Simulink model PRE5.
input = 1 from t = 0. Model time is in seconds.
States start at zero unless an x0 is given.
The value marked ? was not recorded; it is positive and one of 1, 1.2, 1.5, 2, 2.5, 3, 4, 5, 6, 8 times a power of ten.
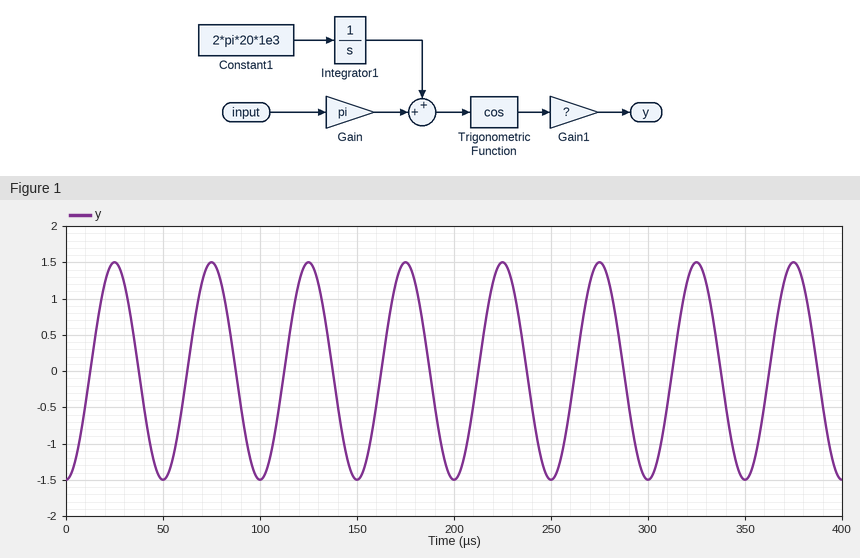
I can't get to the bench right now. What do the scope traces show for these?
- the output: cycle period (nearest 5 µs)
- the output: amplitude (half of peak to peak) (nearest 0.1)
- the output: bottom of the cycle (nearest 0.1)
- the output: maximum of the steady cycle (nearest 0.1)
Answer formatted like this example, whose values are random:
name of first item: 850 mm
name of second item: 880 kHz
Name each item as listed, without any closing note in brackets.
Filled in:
the output: cycle period: 50 µs
the output: amplitude (half of peak to peak): 1.5
the output: bottom of the cycle: -1.5
the output: maximum of the steady cycle: 1.5
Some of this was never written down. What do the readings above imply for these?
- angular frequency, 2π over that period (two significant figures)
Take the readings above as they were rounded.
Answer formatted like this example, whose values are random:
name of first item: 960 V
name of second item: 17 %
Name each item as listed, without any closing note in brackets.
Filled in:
angular frequency, 2π over that period: 0.13 rad/µs
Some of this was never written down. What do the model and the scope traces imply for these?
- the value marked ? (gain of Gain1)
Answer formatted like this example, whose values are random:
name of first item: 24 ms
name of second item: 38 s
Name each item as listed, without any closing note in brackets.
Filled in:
the value marked ?: 1.5
